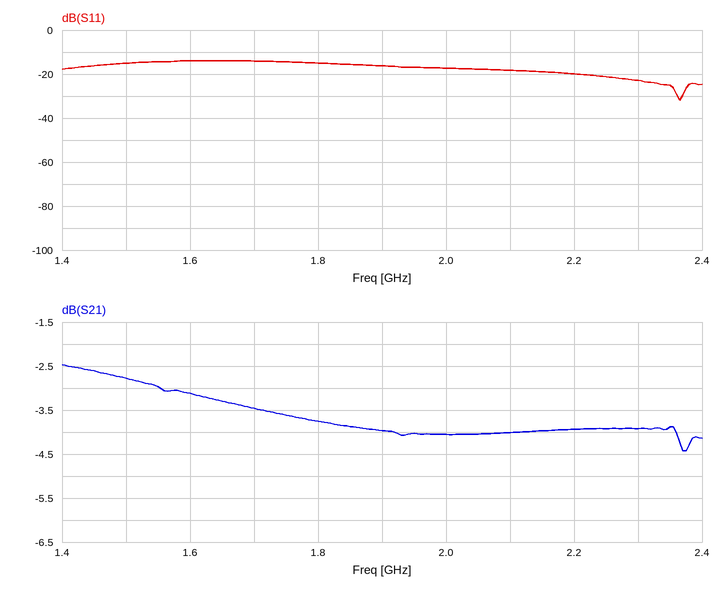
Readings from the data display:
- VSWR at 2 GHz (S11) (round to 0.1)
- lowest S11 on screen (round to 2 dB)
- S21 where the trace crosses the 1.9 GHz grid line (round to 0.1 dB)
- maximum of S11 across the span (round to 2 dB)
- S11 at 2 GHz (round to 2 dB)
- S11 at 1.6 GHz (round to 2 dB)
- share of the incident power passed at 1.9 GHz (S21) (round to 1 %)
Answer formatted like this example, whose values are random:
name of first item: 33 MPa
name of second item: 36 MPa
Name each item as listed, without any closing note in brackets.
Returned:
VSWR at 2 GHz (S11): 1.3
lowest S11 on screen: -32 dB
S21 where the trace crosses the 1.9 GHz grid line: -4.0 dB
maximum of S11 across the span: -14 dB
S11 at 2 GHz: -18 dB
S11 at 1.6 GHz: -14 dB
share of the incident power passed at 1.9 GHz (S21): 40 %
